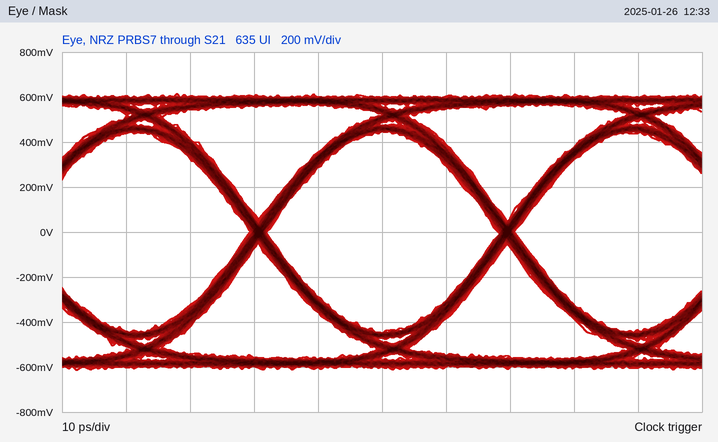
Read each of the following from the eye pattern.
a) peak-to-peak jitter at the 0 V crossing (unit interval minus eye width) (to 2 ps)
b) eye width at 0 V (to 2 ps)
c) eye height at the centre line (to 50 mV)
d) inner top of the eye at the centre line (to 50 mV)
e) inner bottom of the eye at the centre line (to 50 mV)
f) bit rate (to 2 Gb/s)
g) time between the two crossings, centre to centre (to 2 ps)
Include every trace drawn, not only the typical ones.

2 ps
36 ps
900 mV
450 mV
-450 mV
26 Gb/s
38 ps
